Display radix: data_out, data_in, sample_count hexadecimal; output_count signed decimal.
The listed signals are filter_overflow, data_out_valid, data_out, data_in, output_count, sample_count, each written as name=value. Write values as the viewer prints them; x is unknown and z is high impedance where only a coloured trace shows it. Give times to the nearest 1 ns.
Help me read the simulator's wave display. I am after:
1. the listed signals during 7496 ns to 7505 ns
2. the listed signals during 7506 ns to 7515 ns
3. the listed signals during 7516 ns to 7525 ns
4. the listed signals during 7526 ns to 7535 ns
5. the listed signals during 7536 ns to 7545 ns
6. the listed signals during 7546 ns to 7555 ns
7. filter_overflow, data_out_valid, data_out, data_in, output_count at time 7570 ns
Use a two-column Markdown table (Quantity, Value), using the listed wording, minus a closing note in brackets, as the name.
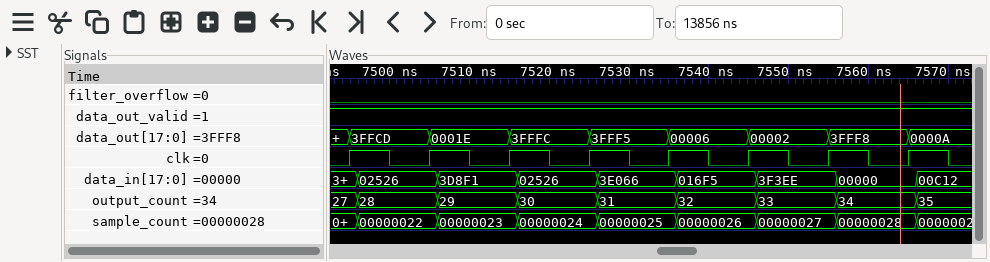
| Quantity | Value |
|---|---|
| the listed signals during 7496 ns to 7505 ns | filter_overflow=0, data_out_valid=1, data_out=3FFCD, data_in=02526, output_count=28, sample_count=00000022 |
| the listed signals during 7506 ns to 7515 ns | filter_overflow=0, data_out_valid=1, data_out=0001E, data_in=3D8F1, output_count=29, sample_count=00000023 |
| the listed signals during 7516 ns to 7525 ns | filter_overflow=0, data_out_valid=1, data_out=3FFFC, data_in=02526, output_count=30, sample_count=00000024 |
| the listed signals during 7526 ns to 7535 ns | filter_overflow=0, data_out_valid=1, data_out=3FFF5, data_in=3E066, output_count=31, sample_count=00000025 |
| the listed signals during 7536 ns to 7545 ns | filter_overflow=0, data_out_valid=1, data_out=00006, data_in=016F5, output_count=32, sample_count=00000026 |
| the listed signals during 7546 ns to 7555 ns | filter_overflow=0, data_out_valid=1, data_out=00002, data_in=3F3EE, output_count=33, sample_count=00000027 |
| filter_overflow, data_out_valid, data_out, data_in, output_count at time 7570 ns | filter_overflow=0, data_out_valid=1, data_out=0000A, data_in=00C12, output_count=35 |
